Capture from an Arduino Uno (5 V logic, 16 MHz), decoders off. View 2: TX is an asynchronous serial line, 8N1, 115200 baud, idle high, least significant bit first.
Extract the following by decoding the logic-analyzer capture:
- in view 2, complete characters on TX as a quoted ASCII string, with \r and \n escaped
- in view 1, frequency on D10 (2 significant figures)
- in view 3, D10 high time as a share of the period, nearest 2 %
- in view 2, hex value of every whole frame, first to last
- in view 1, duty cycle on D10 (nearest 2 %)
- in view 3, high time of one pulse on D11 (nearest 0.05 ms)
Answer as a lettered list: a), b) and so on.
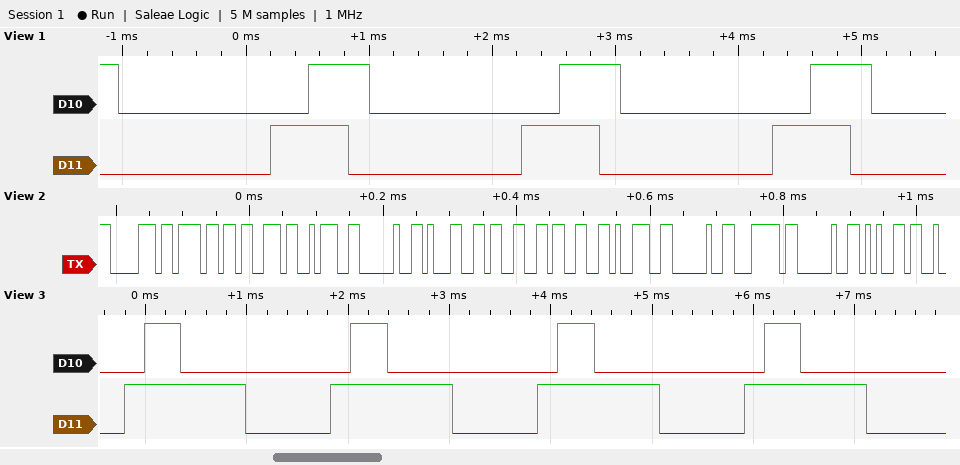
a) "pos: 1339 | e"
b) 490 Hz
c) 18 %
d) 0x70 0x6F 0x73 0x3A 0x20 0x31 0x33 0x33 0x39 0x20 0x7C 0x20 0x65
e) 24 %
f) 1.20 ms
